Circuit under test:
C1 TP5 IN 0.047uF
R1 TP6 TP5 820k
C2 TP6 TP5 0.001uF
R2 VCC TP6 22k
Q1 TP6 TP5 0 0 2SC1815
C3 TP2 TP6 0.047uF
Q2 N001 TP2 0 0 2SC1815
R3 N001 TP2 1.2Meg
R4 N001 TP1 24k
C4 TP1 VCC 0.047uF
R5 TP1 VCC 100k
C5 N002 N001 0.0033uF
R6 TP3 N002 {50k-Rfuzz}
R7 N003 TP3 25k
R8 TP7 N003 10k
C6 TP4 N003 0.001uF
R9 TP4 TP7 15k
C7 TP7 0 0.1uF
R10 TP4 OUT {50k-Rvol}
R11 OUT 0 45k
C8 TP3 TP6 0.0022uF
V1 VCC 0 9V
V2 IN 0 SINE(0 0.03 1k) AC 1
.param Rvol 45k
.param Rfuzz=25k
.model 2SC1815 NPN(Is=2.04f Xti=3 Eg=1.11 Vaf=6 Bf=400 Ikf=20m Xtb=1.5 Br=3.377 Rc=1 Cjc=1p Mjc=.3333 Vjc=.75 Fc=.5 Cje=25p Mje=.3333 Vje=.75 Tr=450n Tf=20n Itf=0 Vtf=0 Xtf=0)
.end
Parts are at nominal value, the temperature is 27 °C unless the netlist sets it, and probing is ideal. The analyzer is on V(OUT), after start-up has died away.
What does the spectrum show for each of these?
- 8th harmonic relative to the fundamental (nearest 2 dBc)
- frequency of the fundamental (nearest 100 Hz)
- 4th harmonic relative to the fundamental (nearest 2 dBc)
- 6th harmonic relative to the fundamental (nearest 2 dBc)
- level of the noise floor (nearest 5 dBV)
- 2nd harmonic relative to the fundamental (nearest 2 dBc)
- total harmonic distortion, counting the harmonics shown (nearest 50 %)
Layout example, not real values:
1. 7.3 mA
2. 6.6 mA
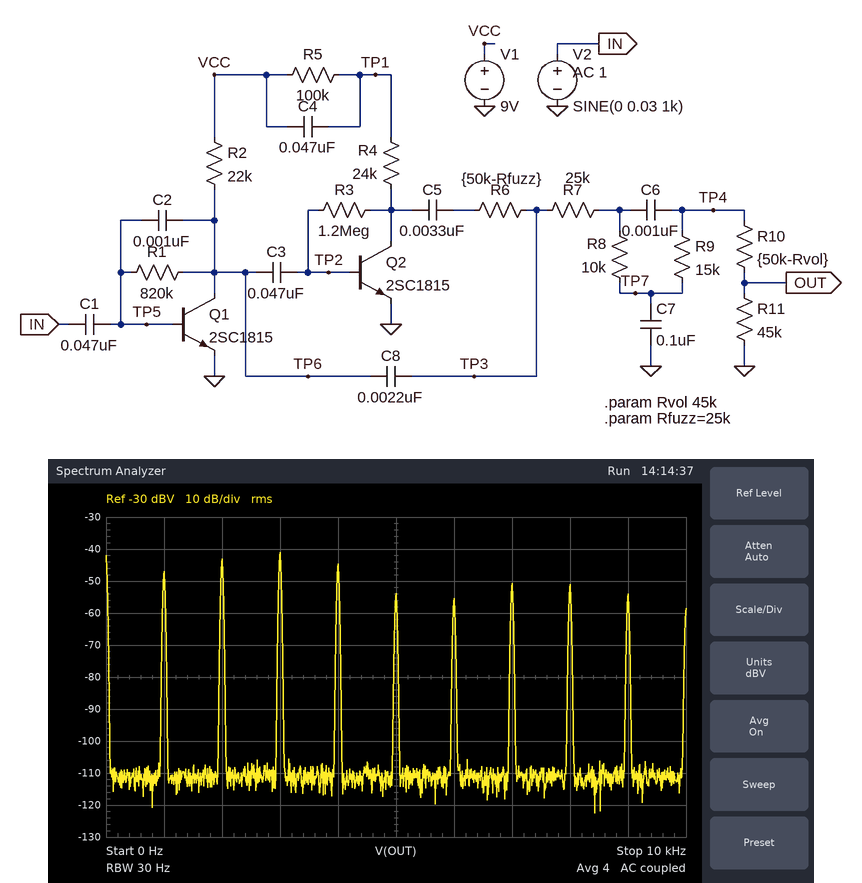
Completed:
1. -4 dBc
2. 1.0 kHz
3. 2 dBc
4. -8 dBc
5. -110 dBV
6. 4 dBc
7. 300 %
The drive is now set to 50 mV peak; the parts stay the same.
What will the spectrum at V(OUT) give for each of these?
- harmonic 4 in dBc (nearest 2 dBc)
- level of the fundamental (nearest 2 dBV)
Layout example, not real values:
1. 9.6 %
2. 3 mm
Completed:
1. 4 dBc
2. -46 dBV
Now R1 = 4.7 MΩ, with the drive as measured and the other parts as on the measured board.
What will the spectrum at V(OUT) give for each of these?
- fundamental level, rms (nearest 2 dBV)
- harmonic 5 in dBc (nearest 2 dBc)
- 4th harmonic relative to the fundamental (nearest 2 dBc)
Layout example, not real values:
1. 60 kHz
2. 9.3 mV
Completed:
1. -46 dBV
2. -12 dBc
3. 0 dBc
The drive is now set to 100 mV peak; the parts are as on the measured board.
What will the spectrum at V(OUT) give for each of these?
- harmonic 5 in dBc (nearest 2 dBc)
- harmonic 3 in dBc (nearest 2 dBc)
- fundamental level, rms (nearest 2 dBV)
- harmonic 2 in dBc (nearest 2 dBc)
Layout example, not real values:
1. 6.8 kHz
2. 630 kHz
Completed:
1. -6 dBc
2. 4 dBc
3. -42 dBV
4. -2 dBc
